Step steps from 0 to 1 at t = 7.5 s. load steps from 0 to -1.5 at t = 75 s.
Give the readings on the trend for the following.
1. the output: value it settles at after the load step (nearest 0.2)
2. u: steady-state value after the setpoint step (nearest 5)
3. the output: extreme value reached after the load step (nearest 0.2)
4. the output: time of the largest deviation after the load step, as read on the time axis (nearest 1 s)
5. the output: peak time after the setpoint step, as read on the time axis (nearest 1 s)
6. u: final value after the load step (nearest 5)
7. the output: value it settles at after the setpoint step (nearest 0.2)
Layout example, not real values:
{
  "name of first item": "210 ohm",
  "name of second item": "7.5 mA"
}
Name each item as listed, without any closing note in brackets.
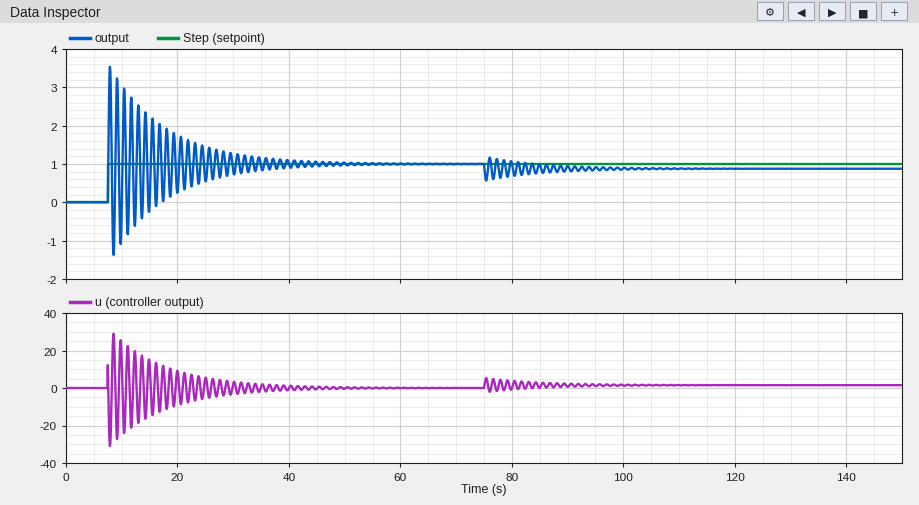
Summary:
{
  "the output: value it settles at after the load step": "0.8",
  "u: steady-state value after the setpoint step": "0",
  "the output: extreme value reached after the load step": "0.6",
  "the output: time of the largest deviation after the load step, as read on the time axis": "75 s",
  "the output: peak time after the setpoint step, as read on the time axis": "8 s",
  "u: final value after the load step": "0",
  "the output: value it settles at after the setpoint step": "1.0"
}
